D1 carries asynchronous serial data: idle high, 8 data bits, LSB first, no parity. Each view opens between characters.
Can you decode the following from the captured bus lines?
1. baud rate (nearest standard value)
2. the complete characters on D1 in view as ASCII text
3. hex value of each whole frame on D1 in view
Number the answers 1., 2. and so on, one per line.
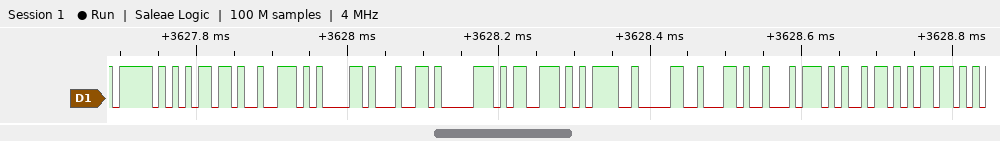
1. 115200 baud
2. "_mradps=0,tim"
3. 5F, 6D, 72, 61, 64, 70, 73, 3D, 30, 2C, 74, 69, 6D
